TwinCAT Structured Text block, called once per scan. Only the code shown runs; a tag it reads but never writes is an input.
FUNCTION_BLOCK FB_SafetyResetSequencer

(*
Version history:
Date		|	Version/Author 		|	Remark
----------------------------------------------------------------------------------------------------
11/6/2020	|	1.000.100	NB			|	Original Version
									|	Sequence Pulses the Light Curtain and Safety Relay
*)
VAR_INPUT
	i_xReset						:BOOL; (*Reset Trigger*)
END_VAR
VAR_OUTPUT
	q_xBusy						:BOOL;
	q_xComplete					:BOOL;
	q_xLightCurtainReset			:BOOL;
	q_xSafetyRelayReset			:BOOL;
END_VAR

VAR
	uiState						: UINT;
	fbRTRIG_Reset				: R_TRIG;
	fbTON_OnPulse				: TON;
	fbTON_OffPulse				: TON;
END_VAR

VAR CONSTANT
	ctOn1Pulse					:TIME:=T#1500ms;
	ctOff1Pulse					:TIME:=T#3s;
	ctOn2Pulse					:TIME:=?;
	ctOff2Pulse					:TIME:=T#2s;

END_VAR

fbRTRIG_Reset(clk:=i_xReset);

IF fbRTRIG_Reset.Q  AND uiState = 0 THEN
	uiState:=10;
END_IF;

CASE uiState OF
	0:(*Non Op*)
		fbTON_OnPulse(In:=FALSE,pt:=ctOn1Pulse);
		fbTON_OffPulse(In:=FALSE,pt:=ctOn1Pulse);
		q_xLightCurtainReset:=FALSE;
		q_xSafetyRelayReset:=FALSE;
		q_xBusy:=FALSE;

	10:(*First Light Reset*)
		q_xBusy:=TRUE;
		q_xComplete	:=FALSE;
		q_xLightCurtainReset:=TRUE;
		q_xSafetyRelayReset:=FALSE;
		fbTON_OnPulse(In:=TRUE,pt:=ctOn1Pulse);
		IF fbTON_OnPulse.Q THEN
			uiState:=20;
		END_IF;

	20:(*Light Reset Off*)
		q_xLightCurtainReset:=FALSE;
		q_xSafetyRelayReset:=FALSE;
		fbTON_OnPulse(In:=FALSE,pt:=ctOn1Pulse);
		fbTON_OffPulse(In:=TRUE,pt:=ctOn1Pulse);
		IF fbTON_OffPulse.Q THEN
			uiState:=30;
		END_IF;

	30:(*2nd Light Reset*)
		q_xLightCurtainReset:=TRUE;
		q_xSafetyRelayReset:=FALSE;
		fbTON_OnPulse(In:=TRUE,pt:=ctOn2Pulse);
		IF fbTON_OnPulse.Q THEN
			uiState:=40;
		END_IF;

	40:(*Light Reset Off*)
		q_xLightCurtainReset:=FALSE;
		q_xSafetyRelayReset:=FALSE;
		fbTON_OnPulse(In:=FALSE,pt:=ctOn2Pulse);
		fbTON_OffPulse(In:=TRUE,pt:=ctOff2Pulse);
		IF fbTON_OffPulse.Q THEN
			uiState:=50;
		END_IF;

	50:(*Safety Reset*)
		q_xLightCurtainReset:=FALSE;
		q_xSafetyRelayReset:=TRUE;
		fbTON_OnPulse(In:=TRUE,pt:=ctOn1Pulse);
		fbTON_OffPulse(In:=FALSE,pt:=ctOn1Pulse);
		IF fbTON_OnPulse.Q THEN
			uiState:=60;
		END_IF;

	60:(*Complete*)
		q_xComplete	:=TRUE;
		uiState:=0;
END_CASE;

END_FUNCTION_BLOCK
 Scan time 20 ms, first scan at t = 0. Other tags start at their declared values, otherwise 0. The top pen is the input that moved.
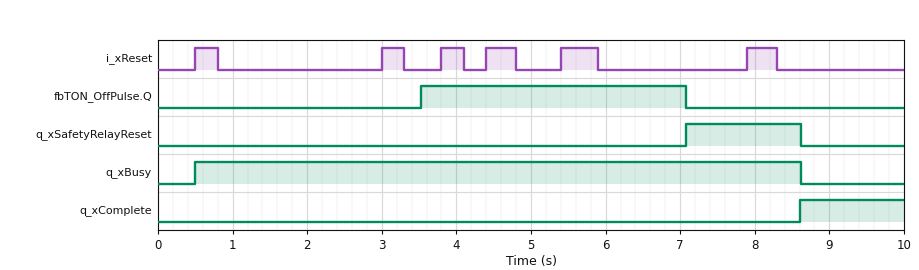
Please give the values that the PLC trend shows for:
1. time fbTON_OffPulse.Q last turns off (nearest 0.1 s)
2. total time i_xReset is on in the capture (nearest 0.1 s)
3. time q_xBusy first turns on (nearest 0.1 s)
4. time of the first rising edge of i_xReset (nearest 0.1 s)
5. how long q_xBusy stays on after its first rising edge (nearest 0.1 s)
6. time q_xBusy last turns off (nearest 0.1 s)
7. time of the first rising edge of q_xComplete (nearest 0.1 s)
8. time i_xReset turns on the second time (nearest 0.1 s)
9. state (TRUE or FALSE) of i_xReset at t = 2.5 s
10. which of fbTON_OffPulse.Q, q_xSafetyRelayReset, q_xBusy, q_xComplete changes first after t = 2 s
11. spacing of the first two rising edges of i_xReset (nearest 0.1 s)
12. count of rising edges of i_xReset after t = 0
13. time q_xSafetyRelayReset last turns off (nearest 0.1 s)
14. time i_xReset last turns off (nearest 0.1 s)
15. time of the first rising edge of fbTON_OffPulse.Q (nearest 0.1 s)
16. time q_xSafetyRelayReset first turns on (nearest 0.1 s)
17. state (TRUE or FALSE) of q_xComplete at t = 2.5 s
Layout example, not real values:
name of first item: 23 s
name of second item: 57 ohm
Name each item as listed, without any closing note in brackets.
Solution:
time fbTON_OffPulse.Q last turns off: 7.1 s
total time i_xReset is on in the capture: 2.2 s
time q_xBusy first turns on: 0.5 s
time of the first rising edge of i_xReset: 0.5 s
how long q_xBusy stays on after its first rising edge: 8.1 s
time q_xBusy last turns off: 8.6 s
time of the first rising edge of q_xComplete: 8.6 s
time i_xReset turns on the second time: 3.0 s
state (TRUE or FALSE) of i_xReset at t = 2.5 s: FALSE
which of fbTON_OffPulse.Q, q_xSafetyRelayReset, q_xBusy, q_xComplete changes first after t = 2 s: fbTON_OffPulse.Q
spacing of the first two rising edges of i_xReset: 2.5 s
count of rising edges of i_xReset after t = 0: 6
time q_xSafetyRelayReset last turns off: 8.6 s
time i_xReset last turns off: 8.3 s
time of the first rising edge of fbTON_OffPulse.Q: 3.5 s
time q_xSafetyRelayReset first turns on: 7.1 s
state (TRUE or FALSE) of q_xComplete at t = 2.5 s: FALSE
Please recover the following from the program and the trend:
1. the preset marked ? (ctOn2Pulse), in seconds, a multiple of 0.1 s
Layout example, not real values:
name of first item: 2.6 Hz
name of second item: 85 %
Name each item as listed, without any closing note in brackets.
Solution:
the preset marked ? (ctOn2Pulse), in seconds, a multiple of 0.1 s: 3.5 s
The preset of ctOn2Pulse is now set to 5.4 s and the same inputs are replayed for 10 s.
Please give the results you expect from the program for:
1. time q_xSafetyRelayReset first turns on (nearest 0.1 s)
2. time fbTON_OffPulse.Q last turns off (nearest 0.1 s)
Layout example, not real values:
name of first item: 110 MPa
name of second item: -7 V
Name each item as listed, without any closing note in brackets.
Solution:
time q_xSafetyRelayReset first turns on: 9.0 s
time fbTON_OffPulse.Q last turns off: 9.0 s
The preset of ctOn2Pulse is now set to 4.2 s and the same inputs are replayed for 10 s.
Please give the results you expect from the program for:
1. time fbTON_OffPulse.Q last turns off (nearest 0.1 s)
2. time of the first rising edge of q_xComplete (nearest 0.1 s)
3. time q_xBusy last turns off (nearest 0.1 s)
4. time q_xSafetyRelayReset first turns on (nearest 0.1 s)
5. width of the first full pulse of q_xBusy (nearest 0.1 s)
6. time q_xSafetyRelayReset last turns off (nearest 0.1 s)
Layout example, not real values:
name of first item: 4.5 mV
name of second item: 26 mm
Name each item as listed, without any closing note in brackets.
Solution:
time fbTON_OffPulse.Q last turns off: 7.8 s
time of the first rising edge of q_xComplete: 9.3 s
time q_xBusy last turns off: 9.3 s
time q_xSafetyRelayReset first turns on: 7.8 s
width of the first full pulse of q_xBusy: 8.8 s
time q_xSafetyRelayReset last turns off: 9.3 s
